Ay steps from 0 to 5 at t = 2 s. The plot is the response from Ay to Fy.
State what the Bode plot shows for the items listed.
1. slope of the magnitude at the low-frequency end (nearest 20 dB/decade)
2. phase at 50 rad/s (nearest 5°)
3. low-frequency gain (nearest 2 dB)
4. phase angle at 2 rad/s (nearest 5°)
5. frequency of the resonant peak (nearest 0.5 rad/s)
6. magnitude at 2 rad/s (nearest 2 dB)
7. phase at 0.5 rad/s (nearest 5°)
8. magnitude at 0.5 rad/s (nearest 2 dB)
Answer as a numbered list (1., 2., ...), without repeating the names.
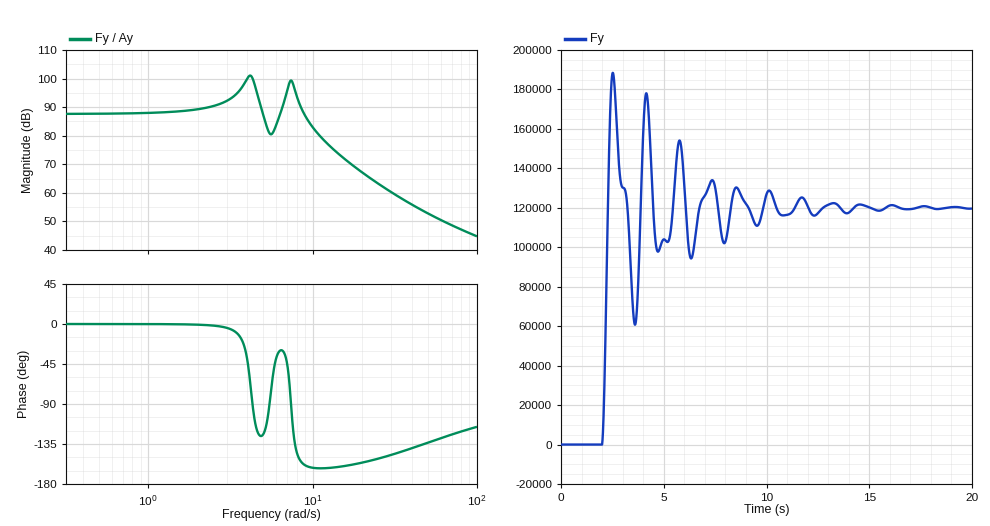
1. 0 dB/decade
2. -135°
3. 88 dB
4. 0°
5. 4.0 rad/s
6. 90 dB
7. 0°
8. 88 dB
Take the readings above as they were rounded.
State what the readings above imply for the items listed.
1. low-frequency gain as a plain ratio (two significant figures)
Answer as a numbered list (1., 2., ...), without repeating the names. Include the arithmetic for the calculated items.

1. 10^(88 / 20) = 25000
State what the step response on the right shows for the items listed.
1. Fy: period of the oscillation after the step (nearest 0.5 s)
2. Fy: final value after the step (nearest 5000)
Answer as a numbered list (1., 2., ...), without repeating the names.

1. 1.5 s
2. 120000
